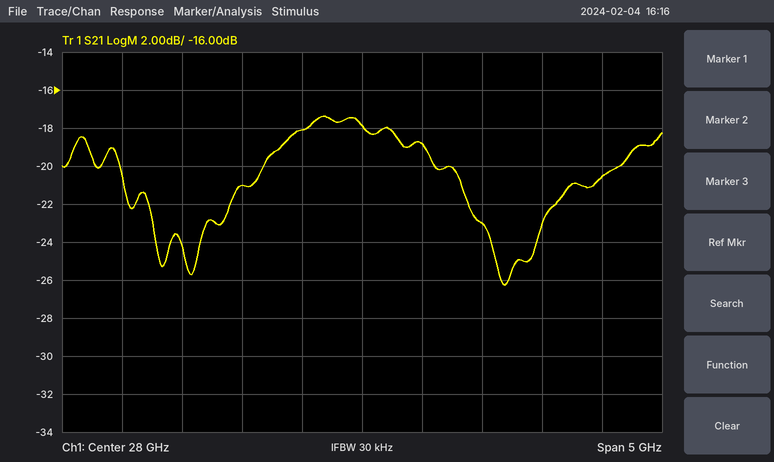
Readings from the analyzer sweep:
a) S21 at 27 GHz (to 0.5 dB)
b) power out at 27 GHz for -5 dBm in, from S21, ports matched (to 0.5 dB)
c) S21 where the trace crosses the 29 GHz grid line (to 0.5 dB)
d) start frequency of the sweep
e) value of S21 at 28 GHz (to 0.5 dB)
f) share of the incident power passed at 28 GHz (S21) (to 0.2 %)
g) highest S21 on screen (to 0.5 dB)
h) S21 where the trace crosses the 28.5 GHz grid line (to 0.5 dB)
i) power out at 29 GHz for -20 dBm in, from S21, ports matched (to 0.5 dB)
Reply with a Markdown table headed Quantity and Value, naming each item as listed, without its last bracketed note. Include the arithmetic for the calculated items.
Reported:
| Quantity | Value |
|---|---|
| S21 at 27 GHz | -21.0 dB |
| power out at 27 GHz for -5 dBm in, from S21, ports matched | -5 dBm + (-21.0 dB) = -26.0 dBm |
| S21 where the trace crosses the 29 GHz grid line | -23.0 dB |
| start frequency of the sweep | 25.5 GHz |
| value of S21 at 28 GHz | -18.0 dB |
| share of the incident power passed at 28 GHz (S21) | 10^(-18/10) ≈ 1.6 % |
| highest S21 on screen | -17.5 dB |
| S21 where the trace crosses the 28.5 GHz grid line | -19.0 dB |
| power out at 29 GHz for -20 dBm in, from S21, ports matched | -20 dBm + (-23.0 dB) = -43.0 dBm |
